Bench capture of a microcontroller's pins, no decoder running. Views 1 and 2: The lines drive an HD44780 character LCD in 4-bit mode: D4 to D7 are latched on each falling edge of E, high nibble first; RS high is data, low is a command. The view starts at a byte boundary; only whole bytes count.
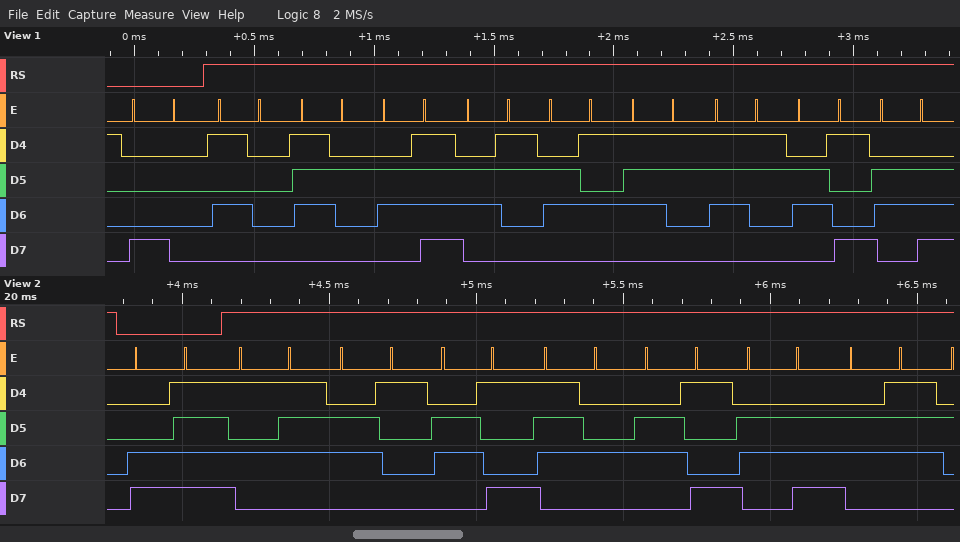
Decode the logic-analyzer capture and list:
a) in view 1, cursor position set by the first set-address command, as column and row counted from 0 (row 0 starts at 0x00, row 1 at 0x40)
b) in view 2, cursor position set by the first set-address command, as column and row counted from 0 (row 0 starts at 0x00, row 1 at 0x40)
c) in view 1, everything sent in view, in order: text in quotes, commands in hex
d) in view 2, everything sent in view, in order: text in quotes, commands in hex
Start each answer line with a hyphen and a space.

- column 0, row 0
- column 15, row 1
- 0x80 "Processin"
- 0xCF "Waiting"
